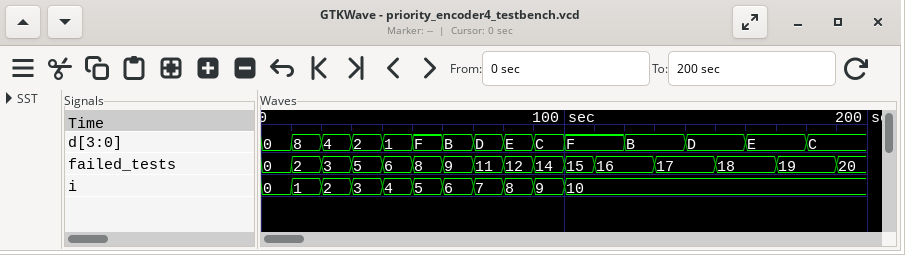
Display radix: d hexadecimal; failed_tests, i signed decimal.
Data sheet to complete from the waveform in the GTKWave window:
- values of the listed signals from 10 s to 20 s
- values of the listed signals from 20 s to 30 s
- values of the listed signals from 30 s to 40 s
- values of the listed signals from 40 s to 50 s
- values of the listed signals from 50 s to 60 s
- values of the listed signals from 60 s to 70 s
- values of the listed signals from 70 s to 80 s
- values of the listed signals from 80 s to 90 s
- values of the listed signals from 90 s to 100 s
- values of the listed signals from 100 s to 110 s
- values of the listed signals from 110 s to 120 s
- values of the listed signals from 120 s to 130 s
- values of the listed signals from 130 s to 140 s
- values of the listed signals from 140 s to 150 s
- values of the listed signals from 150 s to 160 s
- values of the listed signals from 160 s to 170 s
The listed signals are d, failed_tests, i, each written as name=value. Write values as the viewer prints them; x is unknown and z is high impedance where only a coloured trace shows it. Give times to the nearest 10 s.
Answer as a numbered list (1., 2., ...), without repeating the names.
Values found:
1. d=8, failed_tests=2, i=1
2. d=4, failed_tests=3, i=2
3. d=2, failed_tests=5, i=3
4. d=1, failed_tests=6, i=4
5. d=F, failed_tests=8, i=5
6. d=B, failed_tests=9, i=6
7. d=D, failed_tests=11, i=7
8. d=E, failed_tests=12, i=8
9. d=C, failed_tests=14, i=9
10. d=F, failed_tests=15, i=10
11. d=F, failed_tests=16, i=10
12. d=B, failed_tests=16, i=10
13. d=B, failed_tests=17, i=10
14. d=D, failed_tests=17, i=10
15. d=D, failed_tests=18, i=10
16. d=E, failed_tests=18, i=10
